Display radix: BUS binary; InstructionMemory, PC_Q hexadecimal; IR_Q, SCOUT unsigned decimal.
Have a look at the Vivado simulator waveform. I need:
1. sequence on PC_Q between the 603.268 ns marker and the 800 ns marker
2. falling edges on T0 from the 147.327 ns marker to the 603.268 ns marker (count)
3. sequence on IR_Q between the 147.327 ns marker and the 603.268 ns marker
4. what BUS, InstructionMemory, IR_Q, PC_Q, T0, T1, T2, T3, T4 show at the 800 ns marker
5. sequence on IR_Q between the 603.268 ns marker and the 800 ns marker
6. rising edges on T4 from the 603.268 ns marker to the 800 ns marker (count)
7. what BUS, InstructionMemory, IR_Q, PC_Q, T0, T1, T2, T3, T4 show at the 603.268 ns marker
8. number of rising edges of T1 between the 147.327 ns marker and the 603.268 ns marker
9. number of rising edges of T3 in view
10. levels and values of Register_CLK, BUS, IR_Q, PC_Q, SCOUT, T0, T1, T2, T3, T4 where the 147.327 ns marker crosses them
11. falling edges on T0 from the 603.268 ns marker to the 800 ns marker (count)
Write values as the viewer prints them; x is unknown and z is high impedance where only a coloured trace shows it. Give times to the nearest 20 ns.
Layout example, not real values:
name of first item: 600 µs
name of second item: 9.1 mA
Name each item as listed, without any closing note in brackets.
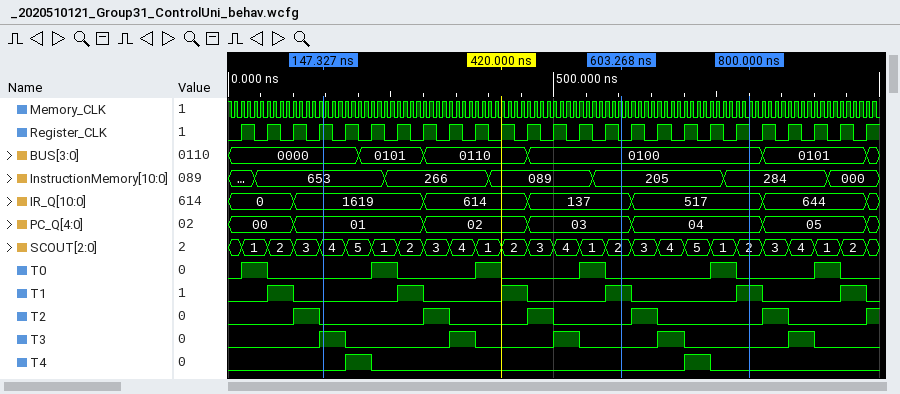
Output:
sequence on PC_Q between the 603.268 ns marker and the 800 ns marker: 03, 04
falling edges on T0 from the 147.327 ns marker to the 603.268 ns marker: 3
sequence on IR_Q between the 147.327 ns marker and the 603.268 ns marker: 1619, 614, 137
what BUS, InstructionMemory, IR_Q, PC_Q, T0, T1, T2, T3, T4 show at the 800 ns marker: BUS=0100, InstructionMemory=284, IR_Q=517, PC_Q=04, T0=0, T1=1, T2=0, T3=0, T4=0
sequence on IR_Q between the 603.268 ns marker and the 800 ns marker: 137, 517
rising edges on T4 from the 603.268 ns marker to the 800 ns marker: 1
what BUS, InstructionMemory, IR_Q, PC_Q, T0, T1, T2, T3, T4 show at the 603.268 ns marker: BUS=0100, InstructionMemory=205, IR_Q=137, PC_Q=03, T0=0, T1=1, T2=0, T3=0, T4=0
number of rising edges of T1 between the 147.327 ns marker and the 603.268 ns marker: 3
number of rising edges of T3 in view: 5
levels and values of Register_CLK, BUS, IR_Q, PC_Q, SCOUT, T0, T1, T2, T3, T4 where the 147.327 ns marker crosses them: Register_CLK=1, BUS=0000, IR_Q=1619, PC_Q=01, SCOUT=4, T0=0, T1=0, T2=0, T3=1, T4=0
falling edges on T0 from the 603.268 ns marker to the 800 ns marker: 1
